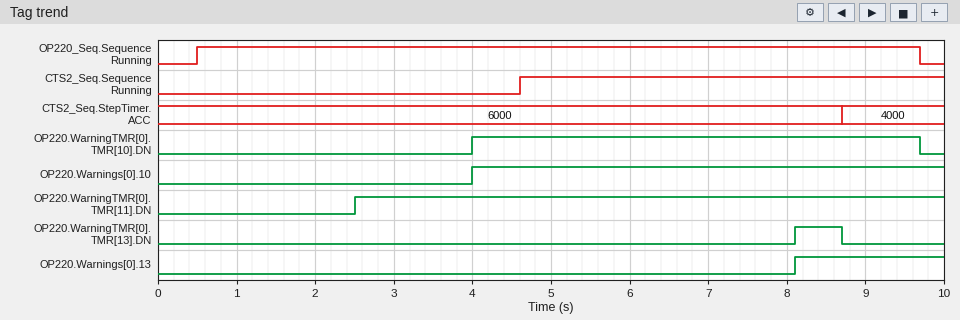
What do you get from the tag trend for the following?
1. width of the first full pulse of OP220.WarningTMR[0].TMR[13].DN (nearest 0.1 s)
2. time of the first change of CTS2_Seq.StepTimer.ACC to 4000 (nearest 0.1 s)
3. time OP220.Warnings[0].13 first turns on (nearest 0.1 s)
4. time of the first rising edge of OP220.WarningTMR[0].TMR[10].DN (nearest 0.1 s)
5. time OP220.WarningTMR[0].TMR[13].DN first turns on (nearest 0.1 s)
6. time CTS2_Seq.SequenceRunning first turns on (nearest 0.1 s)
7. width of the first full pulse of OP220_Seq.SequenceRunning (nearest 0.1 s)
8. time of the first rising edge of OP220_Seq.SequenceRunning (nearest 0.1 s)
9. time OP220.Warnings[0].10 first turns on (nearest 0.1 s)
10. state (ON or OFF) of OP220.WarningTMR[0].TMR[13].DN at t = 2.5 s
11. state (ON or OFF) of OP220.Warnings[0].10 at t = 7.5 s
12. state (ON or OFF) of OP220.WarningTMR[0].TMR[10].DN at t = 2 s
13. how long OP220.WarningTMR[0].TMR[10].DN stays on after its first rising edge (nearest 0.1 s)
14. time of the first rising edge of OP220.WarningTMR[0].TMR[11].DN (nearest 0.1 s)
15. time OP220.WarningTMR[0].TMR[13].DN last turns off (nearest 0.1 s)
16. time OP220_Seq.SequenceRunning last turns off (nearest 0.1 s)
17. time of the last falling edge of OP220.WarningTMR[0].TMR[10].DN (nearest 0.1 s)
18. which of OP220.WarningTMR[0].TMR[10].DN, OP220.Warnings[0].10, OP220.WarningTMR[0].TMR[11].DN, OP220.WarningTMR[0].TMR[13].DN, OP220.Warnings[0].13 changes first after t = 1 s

0.6 s
8.7 s
8.1 s
4.0 s
8.1 s
4.6 s
9.2 s
0.5 s
4.0 s
OFF
ON
OFF
5.7 s
2.5 s
8.7 s
9.7 s
9.7 s
OP220.WarningTMR[0].TMR[11].DN
